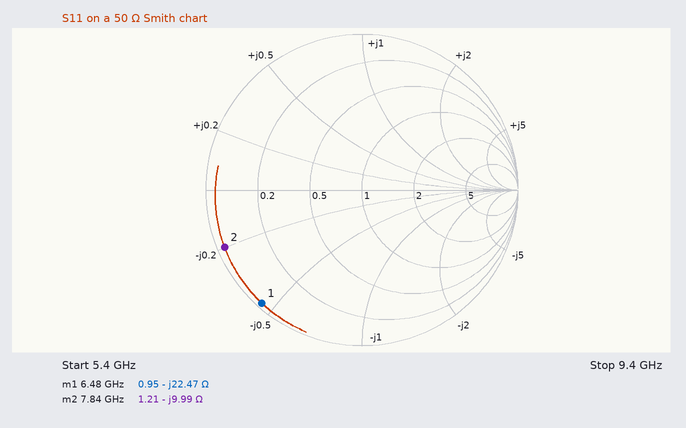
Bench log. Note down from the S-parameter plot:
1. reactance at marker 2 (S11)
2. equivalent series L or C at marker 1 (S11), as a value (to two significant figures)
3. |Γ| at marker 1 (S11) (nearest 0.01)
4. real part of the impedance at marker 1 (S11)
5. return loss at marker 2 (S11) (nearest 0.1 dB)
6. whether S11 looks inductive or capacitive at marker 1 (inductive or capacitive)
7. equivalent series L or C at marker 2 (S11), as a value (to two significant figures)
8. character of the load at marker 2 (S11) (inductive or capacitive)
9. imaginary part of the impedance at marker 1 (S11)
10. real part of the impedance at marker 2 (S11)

-9.99 Ω
1.1 pF
0.97
0.95 Ω
0.4 dB
capacitive
2.0 pF
capacitive
-22.47 Ω
1.21 Ω
